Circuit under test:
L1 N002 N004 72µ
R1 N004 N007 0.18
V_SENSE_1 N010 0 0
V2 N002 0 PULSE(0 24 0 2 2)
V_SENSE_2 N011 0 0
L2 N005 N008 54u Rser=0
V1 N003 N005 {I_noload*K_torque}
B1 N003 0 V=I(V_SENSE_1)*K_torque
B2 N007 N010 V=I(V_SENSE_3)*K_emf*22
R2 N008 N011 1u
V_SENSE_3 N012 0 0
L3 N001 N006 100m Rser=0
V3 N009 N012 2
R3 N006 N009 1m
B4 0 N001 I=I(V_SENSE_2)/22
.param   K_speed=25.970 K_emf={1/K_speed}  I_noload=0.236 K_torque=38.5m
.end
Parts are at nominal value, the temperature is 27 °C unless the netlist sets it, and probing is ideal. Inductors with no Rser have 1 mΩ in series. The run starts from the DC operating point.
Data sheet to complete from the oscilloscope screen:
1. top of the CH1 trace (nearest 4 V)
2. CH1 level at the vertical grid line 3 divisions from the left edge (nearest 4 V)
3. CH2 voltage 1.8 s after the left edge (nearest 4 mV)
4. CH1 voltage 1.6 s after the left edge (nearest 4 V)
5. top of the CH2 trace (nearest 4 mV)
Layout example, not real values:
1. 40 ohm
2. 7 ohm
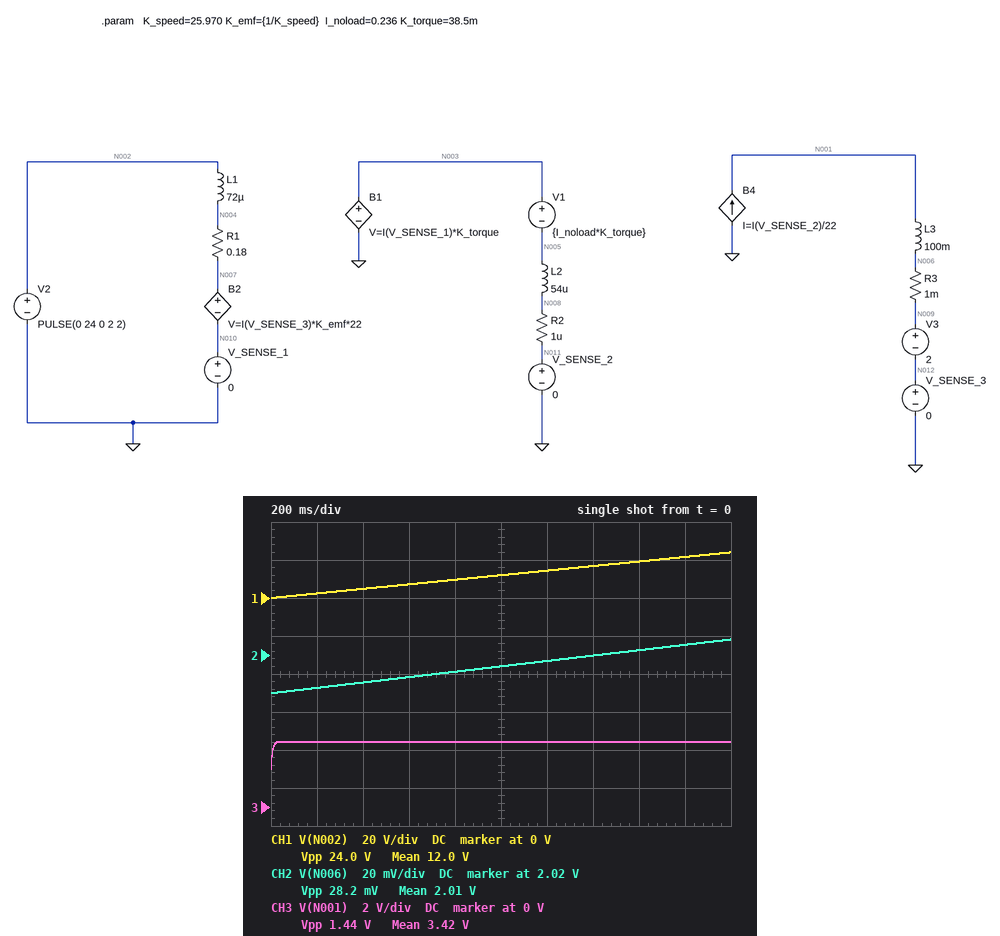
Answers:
1. 24 V
2. 8 V
3. 2.024 V
4. 20 V
5. 2.028 V
